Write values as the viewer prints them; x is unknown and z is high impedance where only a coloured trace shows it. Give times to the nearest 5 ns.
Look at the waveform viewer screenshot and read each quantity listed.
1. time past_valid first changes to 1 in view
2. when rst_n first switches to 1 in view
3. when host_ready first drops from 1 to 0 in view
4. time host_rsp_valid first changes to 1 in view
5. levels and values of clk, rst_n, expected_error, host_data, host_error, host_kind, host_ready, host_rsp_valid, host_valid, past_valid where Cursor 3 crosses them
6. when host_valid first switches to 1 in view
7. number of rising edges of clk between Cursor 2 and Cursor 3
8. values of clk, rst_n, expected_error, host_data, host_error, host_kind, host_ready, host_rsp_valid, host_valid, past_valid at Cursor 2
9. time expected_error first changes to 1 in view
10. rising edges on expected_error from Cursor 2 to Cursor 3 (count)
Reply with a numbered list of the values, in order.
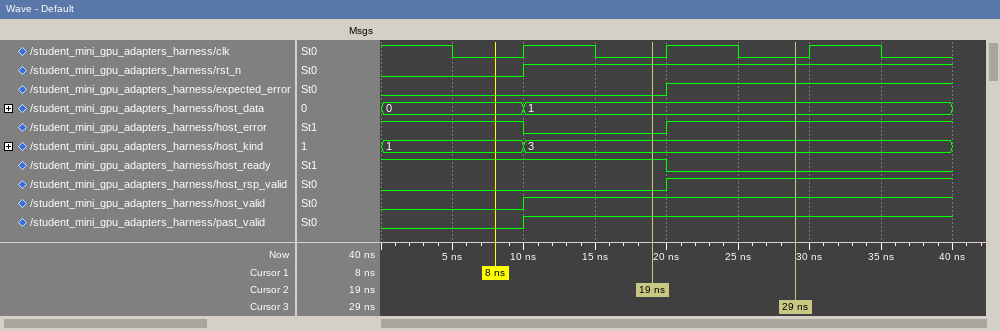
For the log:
1. 10 ns
2. 10 ns
3. 20 ns
4. 20 ns
5. clk=0, rst_n=1, expected_error=1, host_data=1, host_error=1, host_kind=3, host_ready=0, host_rsp_valid=1, host_valid=1, past_valid=1
6. 10 ns
7. 1
8. clk=0, rst_n=1, expected_error=0, host_data=1, host_error=0, host_kind=3, host_ready=1, host_rsp_valid=0, host_valid=1, past_valid=1
9. 20 ns
10. 1
